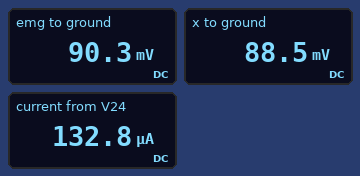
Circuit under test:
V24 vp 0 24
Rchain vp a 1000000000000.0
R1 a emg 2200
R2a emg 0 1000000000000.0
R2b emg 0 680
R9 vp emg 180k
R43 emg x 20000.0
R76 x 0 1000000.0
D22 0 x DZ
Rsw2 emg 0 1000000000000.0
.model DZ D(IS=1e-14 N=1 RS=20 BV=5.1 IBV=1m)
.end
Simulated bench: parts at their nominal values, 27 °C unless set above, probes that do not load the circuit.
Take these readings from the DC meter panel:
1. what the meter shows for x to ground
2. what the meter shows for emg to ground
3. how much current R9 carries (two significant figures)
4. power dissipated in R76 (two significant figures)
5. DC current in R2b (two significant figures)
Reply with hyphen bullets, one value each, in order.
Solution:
- 88.5 mV
- 90.3 mV
- 130 µA
- 7.8 nW
- 130 µA
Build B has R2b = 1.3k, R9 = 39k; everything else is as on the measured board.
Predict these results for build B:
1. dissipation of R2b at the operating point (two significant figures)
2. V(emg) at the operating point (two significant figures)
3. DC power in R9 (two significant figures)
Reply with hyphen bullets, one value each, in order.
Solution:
- 460 µW
- 770 mV
- 14 mW
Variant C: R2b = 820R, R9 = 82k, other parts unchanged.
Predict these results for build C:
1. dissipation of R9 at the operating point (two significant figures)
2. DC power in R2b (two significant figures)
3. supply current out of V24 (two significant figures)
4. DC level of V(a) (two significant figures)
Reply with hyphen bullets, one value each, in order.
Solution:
- 6.9 mW
- 69 µW
- 290 µA
- 240 mV
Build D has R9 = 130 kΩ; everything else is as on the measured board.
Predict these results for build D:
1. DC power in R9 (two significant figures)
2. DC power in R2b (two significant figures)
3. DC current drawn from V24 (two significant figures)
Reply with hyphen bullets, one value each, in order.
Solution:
- 4.4 mW
- 23 µW
- 180 µA
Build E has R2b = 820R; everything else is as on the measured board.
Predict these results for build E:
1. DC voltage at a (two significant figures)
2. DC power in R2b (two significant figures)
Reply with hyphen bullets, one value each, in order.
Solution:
- 110 mV
- 14 µW
